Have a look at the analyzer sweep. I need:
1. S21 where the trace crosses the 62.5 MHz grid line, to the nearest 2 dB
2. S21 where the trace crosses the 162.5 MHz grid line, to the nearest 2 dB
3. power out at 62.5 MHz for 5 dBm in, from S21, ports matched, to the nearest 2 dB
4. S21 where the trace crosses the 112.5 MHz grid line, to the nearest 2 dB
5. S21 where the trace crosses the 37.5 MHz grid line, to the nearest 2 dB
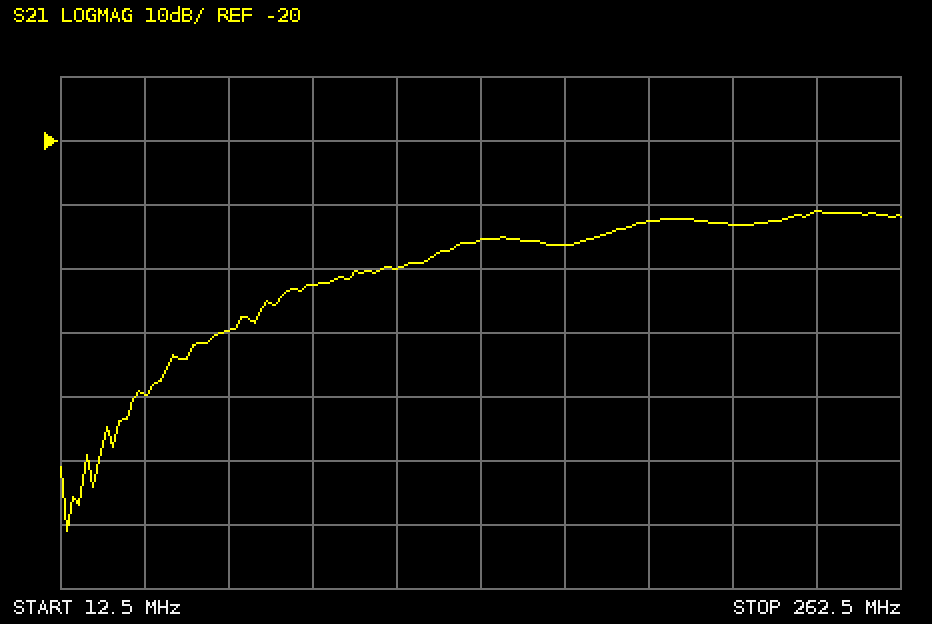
-50 dB
-36 dB
-44 dBm
-40 dB
-60 dB
